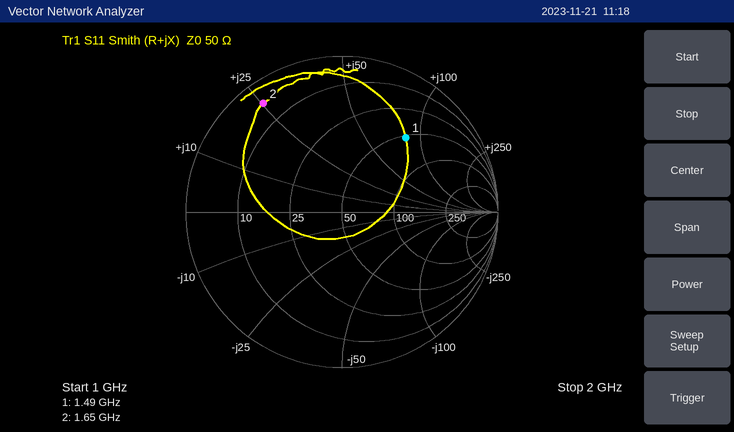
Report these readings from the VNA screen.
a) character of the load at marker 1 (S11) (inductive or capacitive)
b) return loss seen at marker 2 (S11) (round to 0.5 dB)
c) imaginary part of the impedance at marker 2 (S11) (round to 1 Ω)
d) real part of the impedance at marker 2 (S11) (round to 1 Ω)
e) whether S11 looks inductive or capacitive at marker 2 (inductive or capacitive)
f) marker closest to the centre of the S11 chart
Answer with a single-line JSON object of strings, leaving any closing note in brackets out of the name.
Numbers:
{"character of the load at marker 1 (S11)": "inductive", "return loss seen at marker 2 (S11)": "1.5 dB", "imaginary part of the impedance at marker 2 (S11)": "+25 Ω", "real part of the impedance at marker 2 (S11)": "5 Ω", "whether S11 looks inductive or capacitive at marker 2": "inductive", "marker closest to the centre of the S11 chart": "marker 1"}
